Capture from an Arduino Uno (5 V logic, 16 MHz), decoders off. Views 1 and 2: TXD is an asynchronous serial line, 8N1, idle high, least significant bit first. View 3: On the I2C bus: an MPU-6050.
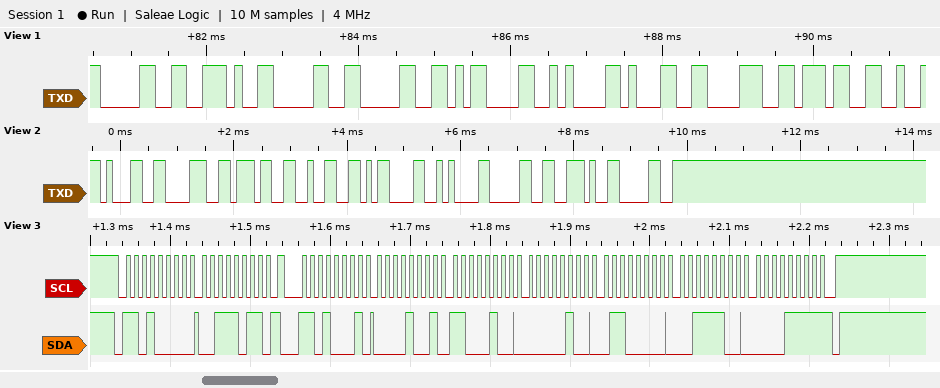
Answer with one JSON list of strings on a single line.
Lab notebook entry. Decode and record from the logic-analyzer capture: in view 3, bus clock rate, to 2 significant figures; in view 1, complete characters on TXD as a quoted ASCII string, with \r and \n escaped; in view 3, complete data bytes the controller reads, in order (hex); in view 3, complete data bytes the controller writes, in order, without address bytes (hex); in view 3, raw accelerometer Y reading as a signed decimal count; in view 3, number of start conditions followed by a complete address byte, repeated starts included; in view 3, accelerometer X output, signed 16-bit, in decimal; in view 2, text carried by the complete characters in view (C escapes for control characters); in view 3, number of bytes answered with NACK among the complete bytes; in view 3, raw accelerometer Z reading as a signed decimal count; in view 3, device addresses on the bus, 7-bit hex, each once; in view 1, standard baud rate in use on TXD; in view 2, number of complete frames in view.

["100 kHz", "\"0.00\\r\\n187\"", "09 C4 04 60 3C 0F", "3B", "1120", "2", "2500", "\"1872\\r\\n0.0\"", "1", "15375", "0x68", "9600 baud", "9"]
